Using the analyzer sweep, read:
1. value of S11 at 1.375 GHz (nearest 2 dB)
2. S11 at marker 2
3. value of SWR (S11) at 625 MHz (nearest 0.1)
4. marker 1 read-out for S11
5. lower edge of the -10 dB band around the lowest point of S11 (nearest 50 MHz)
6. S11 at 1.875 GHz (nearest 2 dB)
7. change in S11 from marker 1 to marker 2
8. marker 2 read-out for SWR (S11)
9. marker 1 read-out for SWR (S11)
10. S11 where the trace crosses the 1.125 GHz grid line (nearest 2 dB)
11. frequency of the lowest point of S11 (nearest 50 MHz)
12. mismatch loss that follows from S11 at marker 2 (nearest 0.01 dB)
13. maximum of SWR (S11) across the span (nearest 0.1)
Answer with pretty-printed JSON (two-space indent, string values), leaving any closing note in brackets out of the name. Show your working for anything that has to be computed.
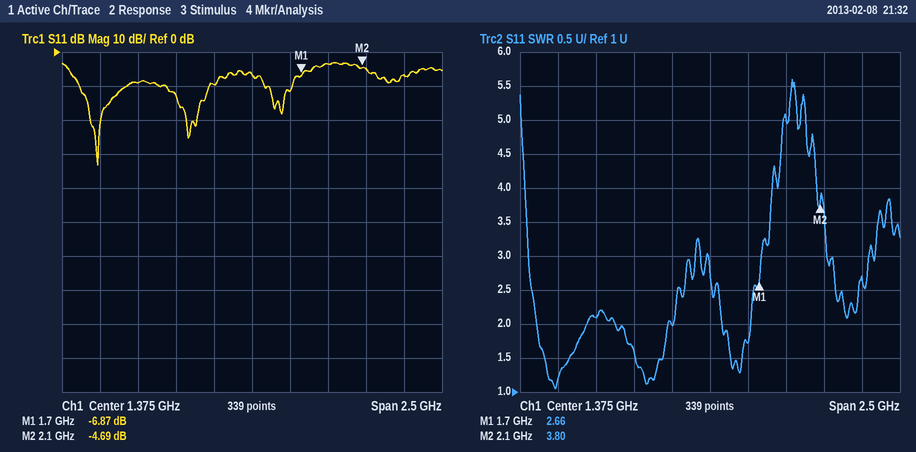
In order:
{
  "value of S11 at 1.375 GHz": "-6 dB",
  "S11 at marker 2": "-4.69 dB",
  "value of SWR (S11) at 625 MHz": "2.1",
  "marker 1 read-out for S11": "-6.87 dB",
  "lower edge of the -10 dB band around the lowest point of S11": "250 MHz",
  "S11 at 1.875 GHz": "-4 dB",
  "change in S11 from marker 1 to marker 2": "-4.69 − (-6.87) = 2.18 dB",
  "marker 2 read-out for SWR": "3.80",
  "marker 1 read-out for SWR": "2.66",
  "S11 where the trace crosses the 1.125 GHz grid line": "-10 dB",
  "frequency of the lowest point of S11": "350 MHz",
  "mismatch loss that follows from S11 at marker 2": "−10 log10(1 − 10^(-4.69/10)) ≈ 1.80 dB",
  "maximum of SWR (S11) across the span": "5.6"
}
